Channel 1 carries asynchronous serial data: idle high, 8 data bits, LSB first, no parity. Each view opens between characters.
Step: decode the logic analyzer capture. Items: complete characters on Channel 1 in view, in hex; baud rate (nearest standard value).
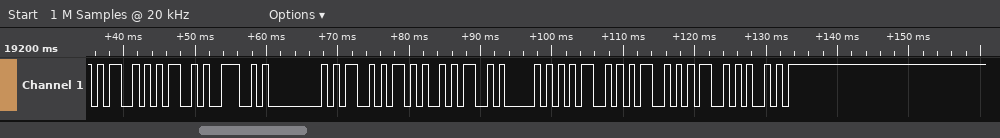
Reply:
4D, 4D, 4E, 00, 4D, 2B, 4D, 50, 4D, 4D, 4D, A9
1200 baud
